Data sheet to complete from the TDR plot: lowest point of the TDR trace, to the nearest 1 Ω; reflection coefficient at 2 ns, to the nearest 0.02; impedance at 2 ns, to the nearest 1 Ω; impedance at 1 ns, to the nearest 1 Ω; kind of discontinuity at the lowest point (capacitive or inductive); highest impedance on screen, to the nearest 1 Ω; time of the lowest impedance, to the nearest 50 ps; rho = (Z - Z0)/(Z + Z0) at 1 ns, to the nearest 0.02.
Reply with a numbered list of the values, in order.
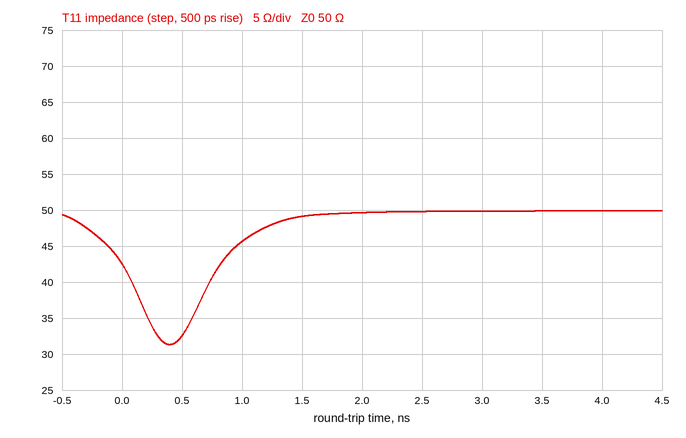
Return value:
1. 31 Ω
2. 0.00
3. 50 Ω
4. 46 Ω
5. capacitive
6. 50 Ω
7. 400 ps
8. -0.04
